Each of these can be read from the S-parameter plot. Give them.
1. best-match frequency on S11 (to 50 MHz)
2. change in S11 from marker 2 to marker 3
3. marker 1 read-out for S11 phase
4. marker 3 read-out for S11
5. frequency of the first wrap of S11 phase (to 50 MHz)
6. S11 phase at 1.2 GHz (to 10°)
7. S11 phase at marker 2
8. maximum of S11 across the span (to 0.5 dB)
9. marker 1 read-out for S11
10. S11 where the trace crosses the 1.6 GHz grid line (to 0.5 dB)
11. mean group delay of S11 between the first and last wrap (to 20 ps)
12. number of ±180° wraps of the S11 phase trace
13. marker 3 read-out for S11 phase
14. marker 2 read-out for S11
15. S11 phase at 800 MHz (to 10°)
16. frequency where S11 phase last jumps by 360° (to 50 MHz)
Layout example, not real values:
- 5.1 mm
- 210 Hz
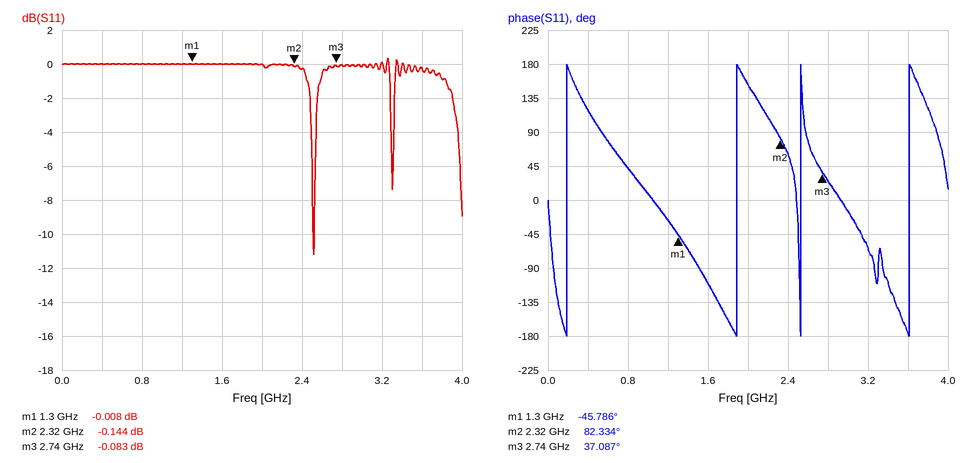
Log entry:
- 2.50 GHz
- 0.061 dB
- -45.786°
- -0.083 dB
- 200 MHz
- -30°
- 82.334°
- 0.5 dB
- -0.008 dB
- 0.0 dB
- 880 ps
- 4
- 37.087°
- -0.144 dB
- 40°
- 3.60 GHz
